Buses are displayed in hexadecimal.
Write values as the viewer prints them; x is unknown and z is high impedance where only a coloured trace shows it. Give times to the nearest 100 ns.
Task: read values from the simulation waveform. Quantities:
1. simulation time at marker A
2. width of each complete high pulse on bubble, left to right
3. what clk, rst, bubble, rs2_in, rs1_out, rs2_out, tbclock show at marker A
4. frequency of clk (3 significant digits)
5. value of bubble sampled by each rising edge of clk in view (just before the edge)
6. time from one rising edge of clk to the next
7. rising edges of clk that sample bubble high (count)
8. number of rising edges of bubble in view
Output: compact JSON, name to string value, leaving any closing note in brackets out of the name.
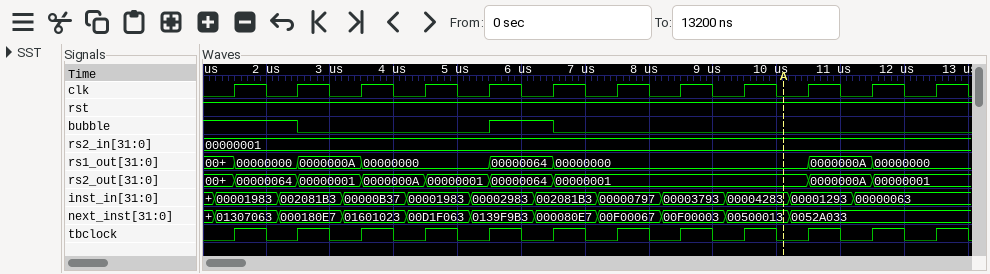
{"simulation time at marker A": "10100 ns", "width of each complete high pulse on bubble, left to right": "1000 ns", "what clk, rst, bubble, rs2_in, rs1_out, rs2_out, tbclock show at marker A": "clk=0, rst=1, bubble=0, rs2_in=00000001, rs1_out=00000000, rs2_out=00000001, tbclock=0", "frequency of clk": "1.00 MHz", "value of bubble sampled by each rising edge of clk in view": "1 1 0 0 0 1 0 0 0 0 0 0", "time from one rising edge of clk to the next": "1000 ns", "rising edges of clk that sample bubble high": "3", "number of rising edges of bubble in view": "1"}
